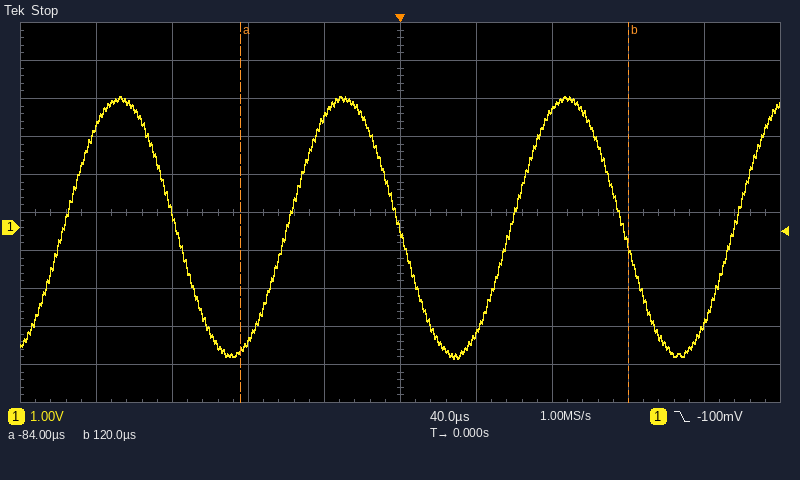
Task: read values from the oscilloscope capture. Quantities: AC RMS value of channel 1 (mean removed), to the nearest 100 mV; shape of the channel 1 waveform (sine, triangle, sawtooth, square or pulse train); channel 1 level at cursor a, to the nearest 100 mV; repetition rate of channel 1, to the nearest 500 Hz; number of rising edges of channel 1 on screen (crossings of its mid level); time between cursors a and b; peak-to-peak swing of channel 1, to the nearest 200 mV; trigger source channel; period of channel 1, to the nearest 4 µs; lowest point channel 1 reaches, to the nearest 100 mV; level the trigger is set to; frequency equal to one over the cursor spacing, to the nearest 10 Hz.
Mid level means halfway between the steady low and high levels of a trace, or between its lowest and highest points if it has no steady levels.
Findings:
2.4 V
sine
-3.2 V
8.5 kHz
4
204 µs
6.8 V
channel 1
116 µs
-3.4 V
-100 mV
4.90 kHz
